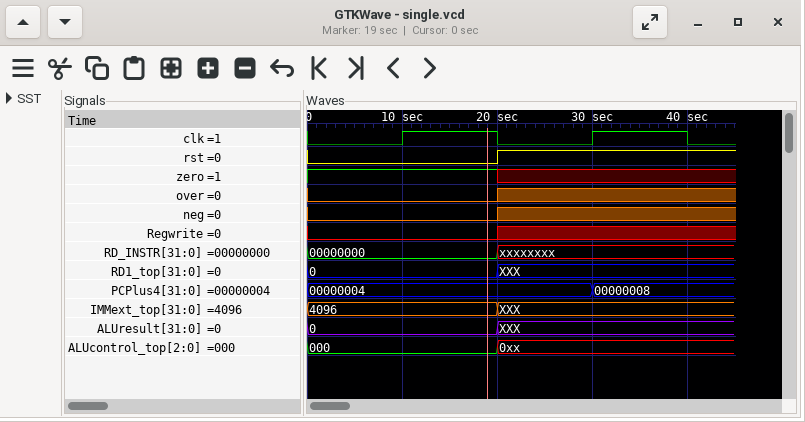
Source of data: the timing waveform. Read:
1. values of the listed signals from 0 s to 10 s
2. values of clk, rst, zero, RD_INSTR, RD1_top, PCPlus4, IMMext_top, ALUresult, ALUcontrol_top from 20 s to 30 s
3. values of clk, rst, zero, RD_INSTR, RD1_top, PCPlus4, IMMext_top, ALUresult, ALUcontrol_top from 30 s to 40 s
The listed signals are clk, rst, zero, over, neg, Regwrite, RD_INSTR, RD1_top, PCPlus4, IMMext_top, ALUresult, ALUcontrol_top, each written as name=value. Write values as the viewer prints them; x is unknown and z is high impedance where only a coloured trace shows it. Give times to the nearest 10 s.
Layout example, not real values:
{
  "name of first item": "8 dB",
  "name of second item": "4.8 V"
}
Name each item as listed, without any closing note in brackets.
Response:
{
  "values of the listed signals from 0 s to 10 s": "clk=0, rst=0, zero=1, over=0, neg=0, Regwrite=0, RD_INSTR=00000000, RD1_top=0, PCPlus4=00000004, IMMext_top=4096, ALUresult=0, ALUcontrol_top=000",
  "values of clk, rst, zero, RD_INSTR, RD1_top, PCPlus4, IMMext_top, ALUresult, ALUcontrol_top from 20 s to 30 s": "clk=0, rst=1, zero=x, RD_INSTR=xxxxxxxx, RD1_top=XXX, PCPlus4=00000004, IMMext_top=XXX, ALUresult=XXX, ALUcontrol_top=0xx",
  "values of clk, rst, zero, RD_INSTR, RD1_top, PCPlus4, IMMext_top, ALUresult, ALUcontrol_top from 30 s to 40 s": "clk=1, rst=1, zero=x, RD_INSTR=xxxxxxxx, RD1_top=XXX, PCPlus4=00000008, IMMext_top=XXX, ALUresult=XXX, ALUcontrol_top=0xx"
}
